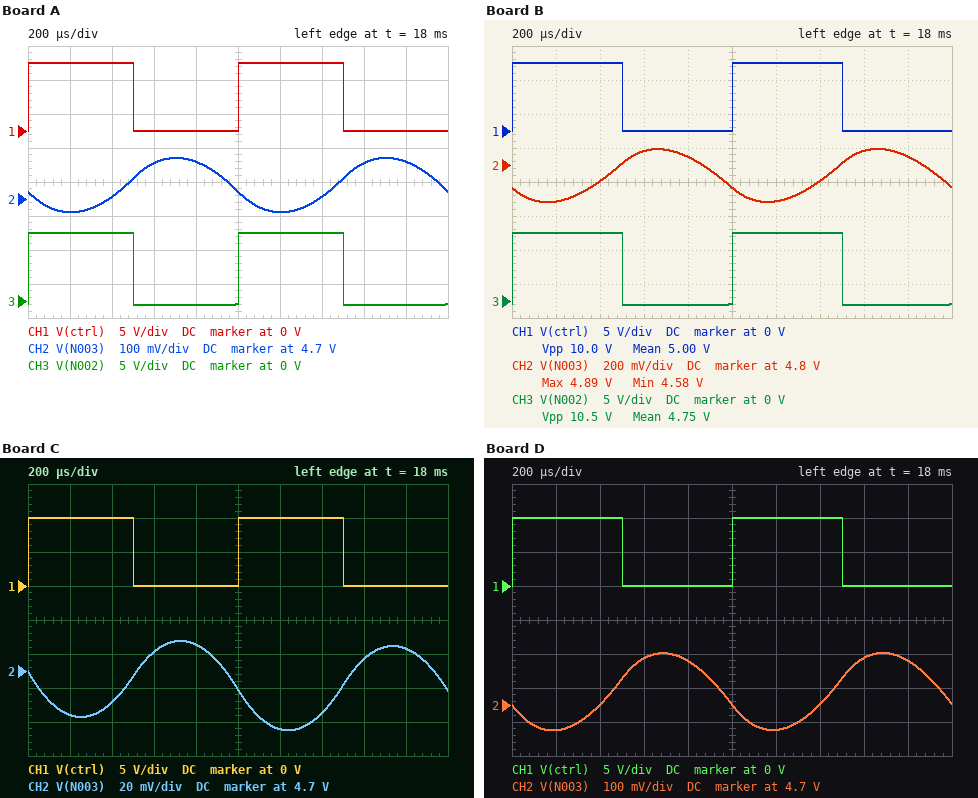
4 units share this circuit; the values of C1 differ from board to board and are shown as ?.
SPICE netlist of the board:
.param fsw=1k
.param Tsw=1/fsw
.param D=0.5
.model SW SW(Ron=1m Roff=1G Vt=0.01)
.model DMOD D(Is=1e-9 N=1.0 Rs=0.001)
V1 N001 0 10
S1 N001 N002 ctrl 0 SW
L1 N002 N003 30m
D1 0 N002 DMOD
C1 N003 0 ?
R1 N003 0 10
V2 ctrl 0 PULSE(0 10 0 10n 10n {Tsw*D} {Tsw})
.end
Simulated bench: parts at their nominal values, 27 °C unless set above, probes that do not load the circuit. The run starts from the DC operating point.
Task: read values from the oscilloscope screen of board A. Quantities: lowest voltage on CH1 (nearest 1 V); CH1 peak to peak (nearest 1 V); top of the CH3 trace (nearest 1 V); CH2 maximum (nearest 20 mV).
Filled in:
0 V
10 V
10 V
4.82 V
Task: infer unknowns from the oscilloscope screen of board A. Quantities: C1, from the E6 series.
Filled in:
68 µF
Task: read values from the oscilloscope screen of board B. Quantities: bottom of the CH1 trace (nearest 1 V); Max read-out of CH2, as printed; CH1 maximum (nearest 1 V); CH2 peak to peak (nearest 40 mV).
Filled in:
0 V
4.89 V
10 V
320 mV
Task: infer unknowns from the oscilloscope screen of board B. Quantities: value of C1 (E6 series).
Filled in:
33 µF
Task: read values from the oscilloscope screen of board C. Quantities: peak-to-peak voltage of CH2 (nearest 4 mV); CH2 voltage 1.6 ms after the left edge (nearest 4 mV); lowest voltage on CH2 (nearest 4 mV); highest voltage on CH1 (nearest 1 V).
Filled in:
52 mV
4.708 V
4.664 V
10 V
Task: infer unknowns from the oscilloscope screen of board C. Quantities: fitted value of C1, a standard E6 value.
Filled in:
220 µF
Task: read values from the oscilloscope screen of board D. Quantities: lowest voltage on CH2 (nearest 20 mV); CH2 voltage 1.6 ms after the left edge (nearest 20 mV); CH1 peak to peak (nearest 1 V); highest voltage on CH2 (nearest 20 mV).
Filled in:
4.62 V
4.84 V
10 V
4.86 V
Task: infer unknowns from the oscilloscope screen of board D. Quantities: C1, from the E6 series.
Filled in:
47 µF
